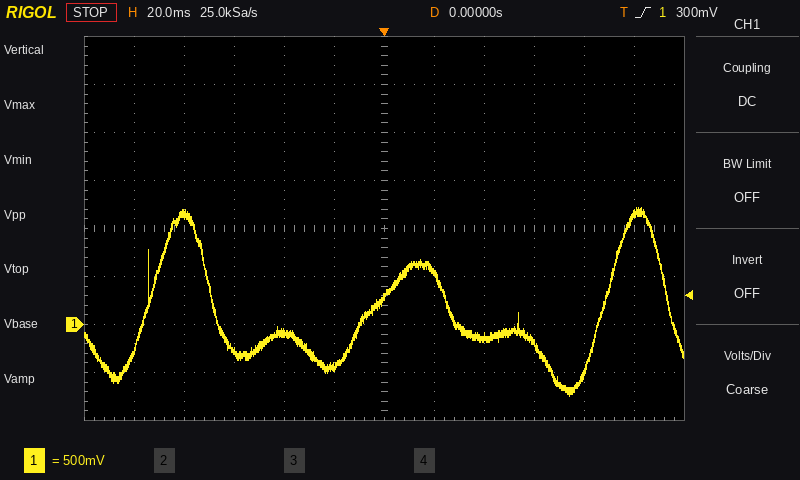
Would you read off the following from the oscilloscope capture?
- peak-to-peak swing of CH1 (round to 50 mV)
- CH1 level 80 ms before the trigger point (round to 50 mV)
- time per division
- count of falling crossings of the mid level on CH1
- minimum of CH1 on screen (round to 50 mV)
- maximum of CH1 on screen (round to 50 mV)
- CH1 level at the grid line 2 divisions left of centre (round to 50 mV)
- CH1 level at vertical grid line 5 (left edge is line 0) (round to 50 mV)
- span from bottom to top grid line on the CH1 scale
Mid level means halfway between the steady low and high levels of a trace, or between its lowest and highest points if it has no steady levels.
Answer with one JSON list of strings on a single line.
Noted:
["1.95 V", "1.15 V", "20 ms", "3", "-750 mV", "1.20 V", "-100 mV", "-450 mV", "4 V"]
